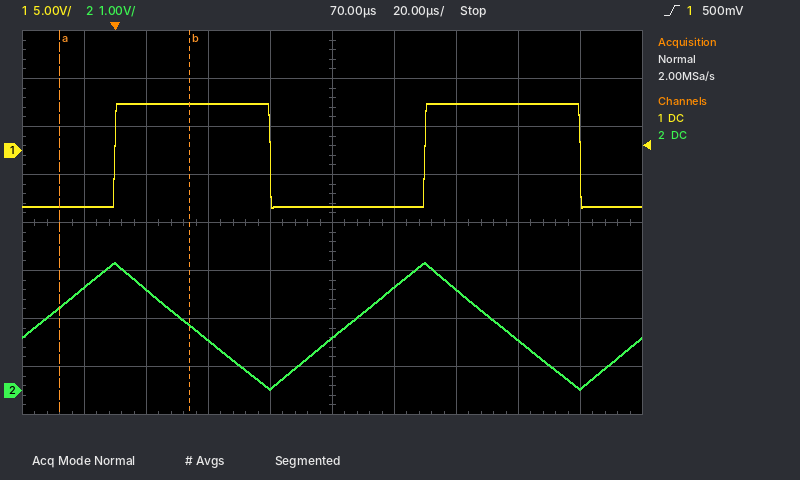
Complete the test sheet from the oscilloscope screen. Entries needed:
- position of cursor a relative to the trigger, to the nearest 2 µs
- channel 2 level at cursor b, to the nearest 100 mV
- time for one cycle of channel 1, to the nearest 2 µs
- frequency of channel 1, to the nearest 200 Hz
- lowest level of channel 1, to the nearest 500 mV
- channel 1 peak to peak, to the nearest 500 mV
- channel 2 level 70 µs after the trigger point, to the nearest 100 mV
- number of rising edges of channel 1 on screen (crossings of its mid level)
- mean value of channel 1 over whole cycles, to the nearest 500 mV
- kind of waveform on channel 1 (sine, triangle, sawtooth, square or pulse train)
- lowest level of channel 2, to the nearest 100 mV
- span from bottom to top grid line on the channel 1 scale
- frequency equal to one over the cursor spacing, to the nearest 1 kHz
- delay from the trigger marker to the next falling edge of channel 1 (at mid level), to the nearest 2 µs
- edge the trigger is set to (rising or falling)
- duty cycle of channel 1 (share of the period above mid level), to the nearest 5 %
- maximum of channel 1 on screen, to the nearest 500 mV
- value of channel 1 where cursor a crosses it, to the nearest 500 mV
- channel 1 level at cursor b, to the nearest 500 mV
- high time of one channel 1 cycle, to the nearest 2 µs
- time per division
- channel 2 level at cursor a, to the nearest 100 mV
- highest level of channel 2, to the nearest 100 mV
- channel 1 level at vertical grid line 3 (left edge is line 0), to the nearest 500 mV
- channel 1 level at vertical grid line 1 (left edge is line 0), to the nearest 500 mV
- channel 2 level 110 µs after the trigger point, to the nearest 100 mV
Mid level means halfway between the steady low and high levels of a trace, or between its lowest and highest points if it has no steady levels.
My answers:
-18 µs
1.4 V
100 µs
10.0 kHz
-6.0 V
11.0 V
1.1 V
2
-500 mV
square
0.0 V
40 V
24 kHz
50 µs
rising
50 %
5.0 V
-6.0 V
5.0 V
50 µs
20 µs
1.7 V
2.7 V
5.0 V
-6.0 V
2.1 V
